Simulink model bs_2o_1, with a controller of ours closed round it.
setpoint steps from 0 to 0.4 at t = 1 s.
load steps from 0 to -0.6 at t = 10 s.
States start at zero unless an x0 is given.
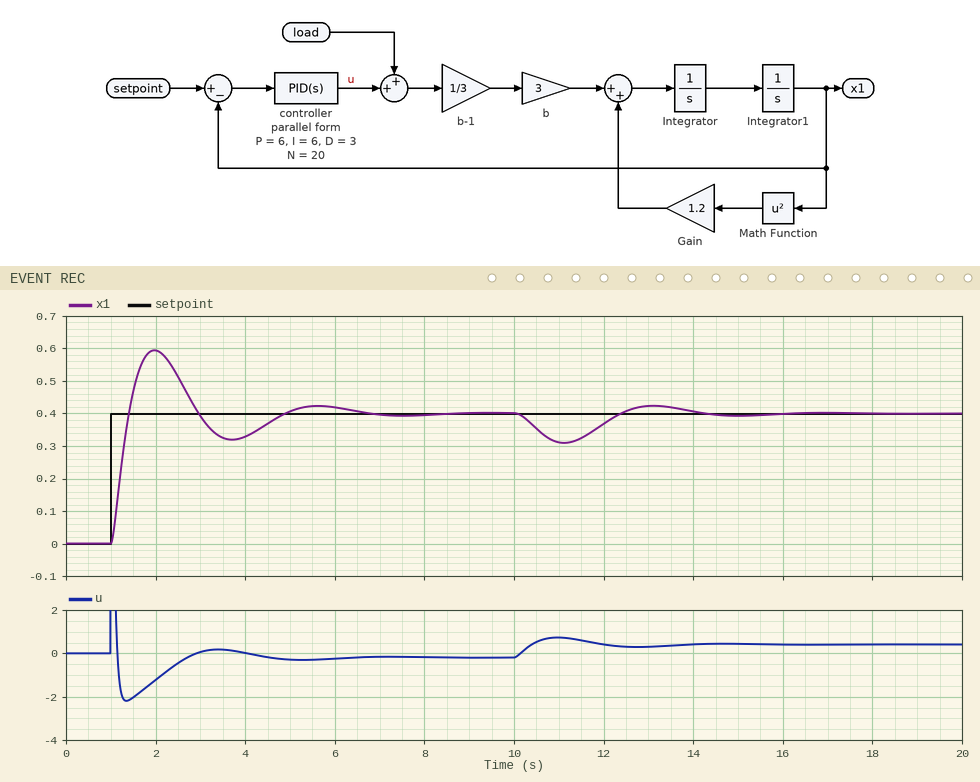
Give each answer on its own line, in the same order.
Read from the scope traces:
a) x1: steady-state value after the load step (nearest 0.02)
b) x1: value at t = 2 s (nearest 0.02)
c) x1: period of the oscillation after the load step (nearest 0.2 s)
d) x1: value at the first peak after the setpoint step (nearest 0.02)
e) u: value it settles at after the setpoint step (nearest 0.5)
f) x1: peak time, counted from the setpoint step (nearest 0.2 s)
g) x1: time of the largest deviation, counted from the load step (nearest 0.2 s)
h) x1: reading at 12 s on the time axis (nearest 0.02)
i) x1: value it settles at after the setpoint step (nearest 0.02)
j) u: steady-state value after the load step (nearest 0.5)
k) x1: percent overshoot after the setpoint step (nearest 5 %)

0.40
0.60
3.8 s
0.60
0.0
1.0 s
1.2 s
0.36
0.40
0.5
50 %
